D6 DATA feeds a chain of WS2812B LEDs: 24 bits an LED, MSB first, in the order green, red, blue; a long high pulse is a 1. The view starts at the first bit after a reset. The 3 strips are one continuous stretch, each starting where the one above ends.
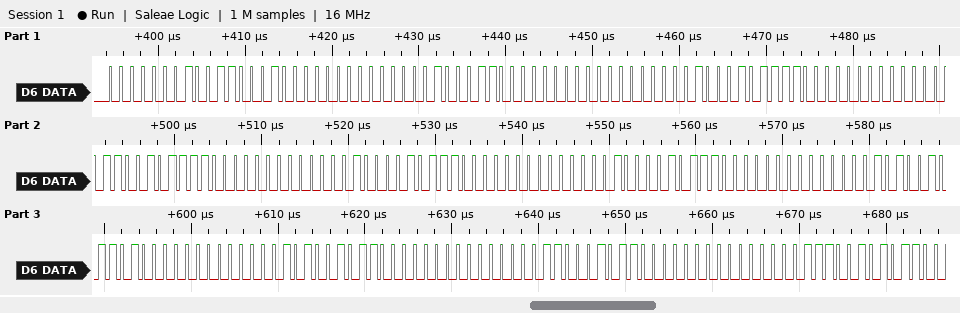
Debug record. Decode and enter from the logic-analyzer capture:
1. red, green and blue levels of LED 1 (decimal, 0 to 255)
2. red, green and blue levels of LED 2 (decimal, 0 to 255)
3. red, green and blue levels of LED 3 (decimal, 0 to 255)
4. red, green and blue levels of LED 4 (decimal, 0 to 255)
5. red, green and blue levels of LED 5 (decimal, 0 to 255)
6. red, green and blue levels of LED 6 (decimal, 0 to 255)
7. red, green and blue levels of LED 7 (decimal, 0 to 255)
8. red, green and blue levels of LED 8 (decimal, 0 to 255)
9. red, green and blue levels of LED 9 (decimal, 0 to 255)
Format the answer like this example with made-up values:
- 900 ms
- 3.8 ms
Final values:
- 49, 1, 0
- 48, 2, 0
- 47, 2, 0
- 47, 3, 0
- 46, 4, 0
- 46, 4, 0
- 45, 5, 0
- 44, 5, 0
- 44, 6, 0
